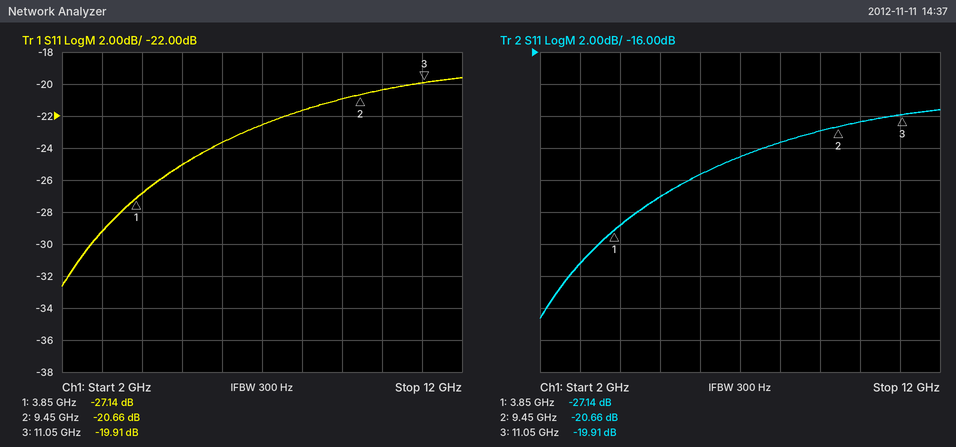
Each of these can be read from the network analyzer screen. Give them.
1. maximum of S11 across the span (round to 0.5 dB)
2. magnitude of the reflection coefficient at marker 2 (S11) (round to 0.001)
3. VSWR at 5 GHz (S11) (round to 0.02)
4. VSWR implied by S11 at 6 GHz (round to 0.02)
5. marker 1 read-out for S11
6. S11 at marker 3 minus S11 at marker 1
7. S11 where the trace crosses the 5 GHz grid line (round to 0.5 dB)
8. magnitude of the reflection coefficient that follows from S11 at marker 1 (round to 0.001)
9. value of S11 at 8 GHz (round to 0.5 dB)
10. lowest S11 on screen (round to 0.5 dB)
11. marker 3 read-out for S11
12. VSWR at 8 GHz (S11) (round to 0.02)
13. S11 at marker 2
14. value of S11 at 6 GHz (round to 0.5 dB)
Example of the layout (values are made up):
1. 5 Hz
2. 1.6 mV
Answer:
1. -19.5 dB
2. 0.093
3. 1.12
4. 1.14
5. -27.14 dB
6. 7.23 dB
7. -25.0 dB
8. 0.044
9. -21.5 dB
10. -32.5 dB
11. -19.91 dB
12. 1.18
13. -20.66 dB
14. -23.5 dB
